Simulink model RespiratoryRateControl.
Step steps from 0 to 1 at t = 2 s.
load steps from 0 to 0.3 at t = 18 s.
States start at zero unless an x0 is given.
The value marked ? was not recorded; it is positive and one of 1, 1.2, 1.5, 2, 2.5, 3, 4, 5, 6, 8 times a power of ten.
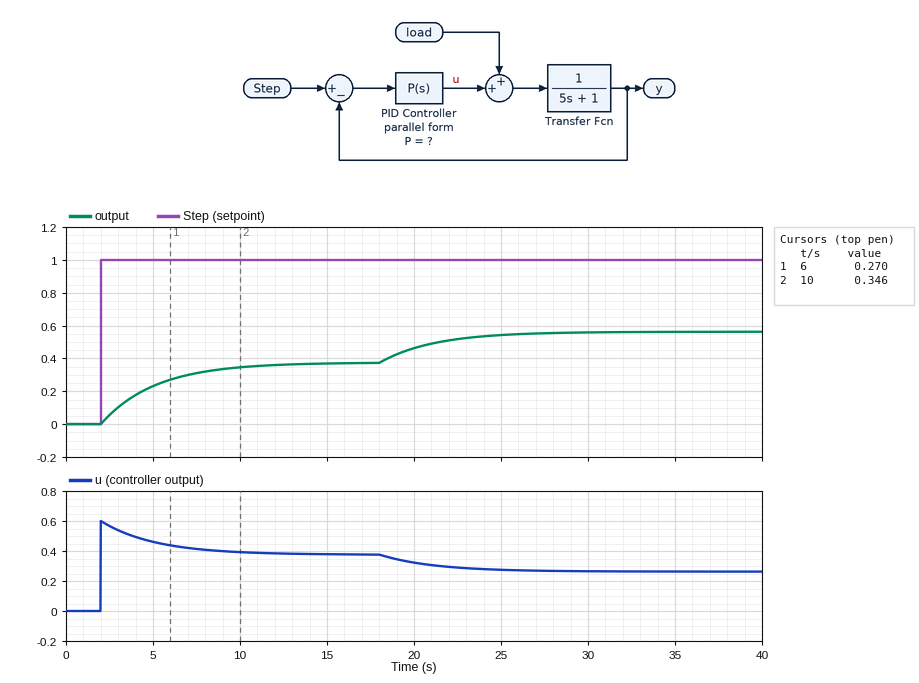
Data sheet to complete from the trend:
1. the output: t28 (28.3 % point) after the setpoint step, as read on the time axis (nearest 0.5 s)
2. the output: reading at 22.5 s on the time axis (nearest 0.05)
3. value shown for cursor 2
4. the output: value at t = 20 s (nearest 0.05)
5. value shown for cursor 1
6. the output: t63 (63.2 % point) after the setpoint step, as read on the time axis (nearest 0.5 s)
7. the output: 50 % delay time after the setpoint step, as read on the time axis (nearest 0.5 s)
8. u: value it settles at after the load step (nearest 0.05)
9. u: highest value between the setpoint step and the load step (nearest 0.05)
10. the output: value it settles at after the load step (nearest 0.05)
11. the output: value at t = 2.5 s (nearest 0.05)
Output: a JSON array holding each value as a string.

["3.0 s", "0.50", "0.346", "0.45", "0.270", "5.0 s", "4.0 s", "0.25", "0.60", "0.55", "0.05"]
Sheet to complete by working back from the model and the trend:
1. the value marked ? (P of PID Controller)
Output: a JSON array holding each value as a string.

["0.6"]
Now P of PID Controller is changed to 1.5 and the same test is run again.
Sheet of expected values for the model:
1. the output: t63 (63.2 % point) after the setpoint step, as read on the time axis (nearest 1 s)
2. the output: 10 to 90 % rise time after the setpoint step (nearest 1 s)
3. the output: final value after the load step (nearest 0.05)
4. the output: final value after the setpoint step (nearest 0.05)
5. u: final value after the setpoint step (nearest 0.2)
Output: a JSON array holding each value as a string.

["4 s", "4 s", "0.70", "0.60", "0.6"]
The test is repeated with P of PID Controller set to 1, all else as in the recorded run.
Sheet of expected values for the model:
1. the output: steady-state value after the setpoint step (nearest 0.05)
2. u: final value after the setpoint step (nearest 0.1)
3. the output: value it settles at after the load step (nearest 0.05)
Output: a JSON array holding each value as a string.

["0.50", "0.5", "0.65"]
